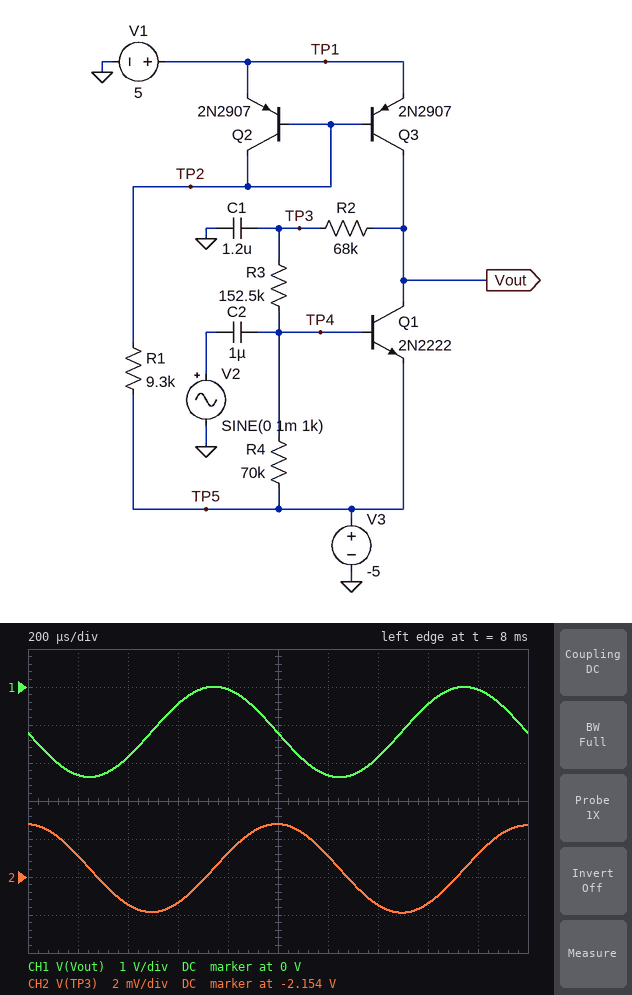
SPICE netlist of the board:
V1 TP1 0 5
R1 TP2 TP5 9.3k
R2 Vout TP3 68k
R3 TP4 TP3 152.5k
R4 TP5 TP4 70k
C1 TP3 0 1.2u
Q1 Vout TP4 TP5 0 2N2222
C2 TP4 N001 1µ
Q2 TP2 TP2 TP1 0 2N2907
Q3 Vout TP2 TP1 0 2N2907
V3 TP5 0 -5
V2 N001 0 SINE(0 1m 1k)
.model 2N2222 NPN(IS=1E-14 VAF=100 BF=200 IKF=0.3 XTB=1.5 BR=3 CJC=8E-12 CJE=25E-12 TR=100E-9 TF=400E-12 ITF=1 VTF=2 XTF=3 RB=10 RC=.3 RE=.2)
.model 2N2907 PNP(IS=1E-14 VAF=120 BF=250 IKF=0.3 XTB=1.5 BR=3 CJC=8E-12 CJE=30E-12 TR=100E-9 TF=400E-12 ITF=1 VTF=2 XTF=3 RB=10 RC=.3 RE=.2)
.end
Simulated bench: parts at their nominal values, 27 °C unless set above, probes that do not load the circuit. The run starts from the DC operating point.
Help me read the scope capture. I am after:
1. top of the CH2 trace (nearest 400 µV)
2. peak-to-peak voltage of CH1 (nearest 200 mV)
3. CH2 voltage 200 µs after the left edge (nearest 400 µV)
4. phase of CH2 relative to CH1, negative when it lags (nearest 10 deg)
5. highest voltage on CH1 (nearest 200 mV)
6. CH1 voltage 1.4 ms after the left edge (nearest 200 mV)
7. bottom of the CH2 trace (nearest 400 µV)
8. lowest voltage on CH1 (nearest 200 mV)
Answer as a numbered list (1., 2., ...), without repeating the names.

1. -2.1512 V
2. 2.4 V
3. -2.1528 V
4. -90 deg
5. 0 V
6. -1.8 V
7. -2.1560 V
8. -2.4 V
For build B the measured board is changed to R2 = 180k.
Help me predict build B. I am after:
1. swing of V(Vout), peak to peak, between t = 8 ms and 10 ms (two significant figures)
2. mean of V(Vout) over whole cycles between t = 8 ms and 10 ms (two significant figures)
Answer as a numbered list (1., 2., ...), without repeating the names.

1. 3.3 V
2. 400 mV
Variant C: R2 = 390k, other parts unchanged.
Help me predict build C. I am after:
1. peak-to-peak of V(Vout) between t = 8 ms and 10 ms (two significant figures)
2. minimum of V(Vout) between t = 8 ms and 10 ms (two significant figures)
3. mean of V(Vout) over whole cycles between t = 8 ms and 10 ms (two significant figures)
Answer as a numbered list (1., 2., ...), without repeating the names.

1. 3.5 V
2. 1.4 V
3. 3.2 V
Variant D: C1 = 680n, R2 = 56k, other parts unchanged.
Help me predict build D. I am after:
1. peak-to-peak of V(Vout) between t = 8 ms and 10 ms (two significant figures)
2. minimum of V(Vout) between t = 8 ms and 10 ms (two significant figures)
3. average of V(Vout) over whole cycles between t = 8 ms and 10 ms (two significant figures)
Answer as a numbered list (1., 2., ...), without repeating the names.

1. 2.2 V
2. -2.5 V
3. -1.4 V
